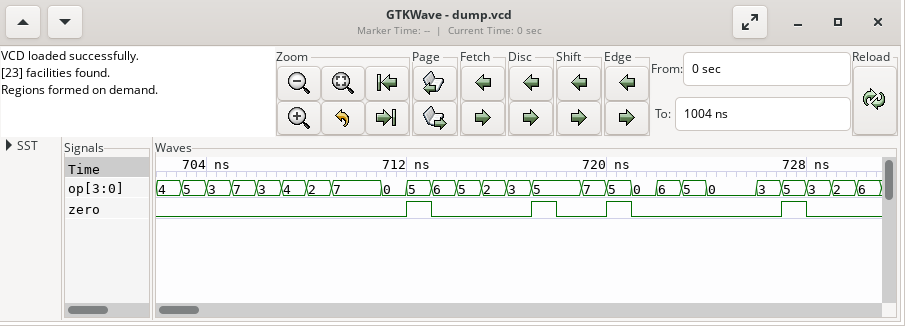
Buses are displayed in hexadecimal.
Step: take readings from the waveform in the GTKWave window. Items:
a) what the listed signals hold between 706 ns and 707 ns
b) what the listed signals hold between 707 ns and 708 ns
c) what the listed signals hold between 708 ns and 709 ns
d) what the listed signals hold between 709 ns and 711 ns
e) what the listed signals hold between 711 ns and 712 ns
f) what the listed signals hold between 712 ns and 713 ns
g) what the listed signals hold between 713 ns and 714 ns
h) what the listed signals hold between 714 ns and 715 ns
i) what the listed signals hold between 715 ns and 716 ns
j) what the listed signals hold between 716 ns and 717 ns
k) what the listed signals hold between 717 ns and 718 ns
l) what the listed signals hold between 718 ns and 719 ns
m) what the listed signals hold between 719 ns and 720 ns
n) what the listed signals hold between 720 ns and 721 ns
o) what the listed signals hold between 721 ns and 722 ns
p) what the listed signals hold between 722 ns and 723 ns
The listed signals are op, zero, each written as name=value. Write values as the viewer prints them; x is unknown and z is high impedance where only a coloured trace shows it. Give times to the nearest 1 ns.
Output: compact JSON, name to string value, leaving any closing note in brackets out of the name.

{"what the listed signals hold between 706 ns and 707 ns": "op=3, zero=0", "what the listed signals hold between 707 ns and 708 ns": "op=4, zero=0", "what the listed signals hold between 708 ns and 709 ns": "op=2, zero=0", "what the listed signals hold between 709 ns and 711 ns": "op=7, zero=0", "what the listed signals hold between 711 ns and 712 ns": "op=0, zero=0", "what the listed signals hold between 712 ns and 713 ns": "op=5, zero=1", "what the listed signals hold between 713 ns and 714 ns": "op=6, zero=0", "what the listed signals hold between 714 ns and 715 ns": "op=5, zero=0", "what the listed signals hold between 715 ns and 716 ns": "op=2, zero=0", "what the listed signals hold between 716 ns and 717 ns": "op=3, zero=0", "what the listed signals hold between 717 ns and 718 ns": "op=5, zero=1", "what the listed signals hold between 718 ns and 719 ns": "op=5, zero=0", "what the listed signals hold between 719 ns and 720 ns": "op=7, zero=0", "what the listed signals hold between 720 ns and 721 ns": "op=5, zero=1", "what the listed signals hold between 721 ns and 722 ns": "op=0, zero=0", "what the listed signals hold between 722 ns and 723 ns": "op=6, zero=0"}
